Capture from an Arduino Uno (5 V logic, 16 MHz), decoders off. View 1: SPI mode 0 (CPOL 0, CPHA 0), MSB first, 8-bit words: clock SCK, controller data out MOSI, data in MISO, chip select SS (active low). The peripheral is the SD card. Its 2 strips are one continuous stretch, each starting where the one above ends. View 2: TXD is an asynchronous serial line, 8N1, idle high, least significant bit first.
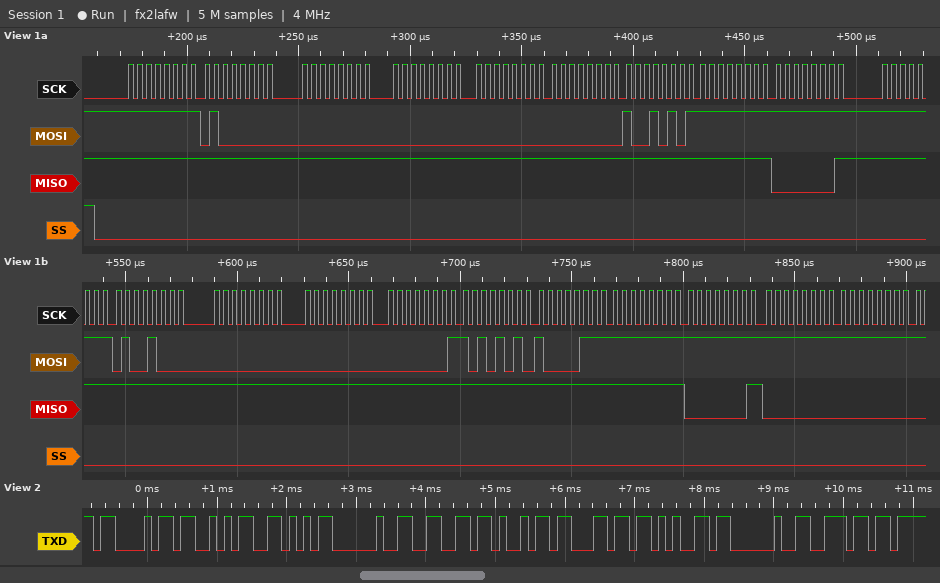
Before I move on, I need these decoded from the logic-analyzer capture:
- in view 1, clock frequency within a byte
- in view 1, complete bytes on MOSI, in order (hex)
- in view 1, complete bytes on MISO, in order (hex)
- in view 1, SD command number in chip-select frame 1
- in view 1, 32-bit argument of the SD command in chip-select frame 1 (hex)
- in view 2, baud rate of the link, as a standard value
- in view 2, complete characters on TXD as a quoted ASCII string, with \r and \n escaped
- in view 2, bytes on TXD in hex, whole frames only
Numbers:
250 kHz
FF 40 00 00 00 00 95 FF FF FF 48 00 00 01 AA 87 FF FF FF FF
FF FF FF FF FF FF FF FF 01 FF FF FF FF FF FF FF FF 01 00 00
CMD0
0x00000000
9600 baud
"CSV file n"
43 53 56 20 66 69 6C 65 20 6E
